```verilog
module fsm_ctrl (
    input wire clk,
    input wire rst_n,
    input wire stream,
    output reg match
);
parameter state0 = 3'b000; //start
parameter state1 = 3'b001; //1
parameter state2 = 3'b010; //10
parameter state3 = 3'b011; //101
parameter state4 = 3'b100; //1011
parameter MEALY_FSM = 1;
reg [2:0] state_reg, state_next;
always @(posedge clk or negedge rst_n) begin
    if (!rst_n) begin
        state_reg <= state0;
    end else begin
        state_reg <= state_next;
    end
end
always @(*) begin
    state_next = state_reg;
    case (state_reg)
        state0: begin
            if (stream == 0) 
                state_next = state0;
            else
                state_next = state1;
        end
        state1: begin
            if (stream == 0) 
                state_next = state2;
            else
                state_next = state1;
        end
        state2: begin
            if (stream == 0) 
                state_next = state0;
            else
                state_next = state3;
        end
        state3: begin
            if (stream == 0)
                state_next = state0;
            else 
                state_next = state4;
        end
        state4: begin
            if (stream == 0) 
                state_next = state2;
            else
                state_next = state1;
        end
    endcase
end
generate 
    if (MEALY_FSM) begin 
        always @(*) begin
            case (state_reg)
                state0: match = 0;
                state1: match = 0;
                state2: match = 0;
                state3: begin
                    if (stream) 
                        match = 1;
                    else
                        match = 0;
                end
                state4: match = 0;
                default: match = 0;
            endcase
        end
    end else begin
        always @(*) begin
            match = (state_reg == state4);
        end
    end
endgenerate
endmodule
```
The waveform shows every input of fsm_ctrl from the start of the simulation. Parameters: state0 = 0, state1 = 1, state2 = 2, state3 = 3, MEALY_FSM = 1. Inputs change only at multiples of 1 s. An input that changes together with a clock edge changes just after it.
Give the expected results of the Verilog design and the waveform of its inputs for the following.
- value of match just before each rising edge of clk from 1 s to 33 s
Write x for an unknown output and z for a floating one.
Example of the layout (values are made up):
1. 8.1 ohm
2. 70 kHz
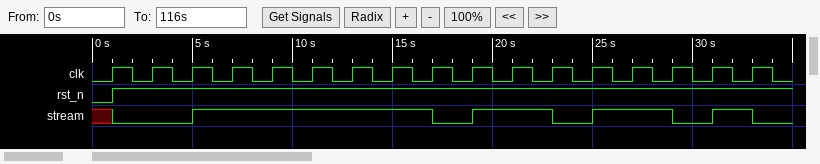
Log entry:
1. 0 0 0 0 0 0 0 0 0 0 0 1 0 0 1 0 0
